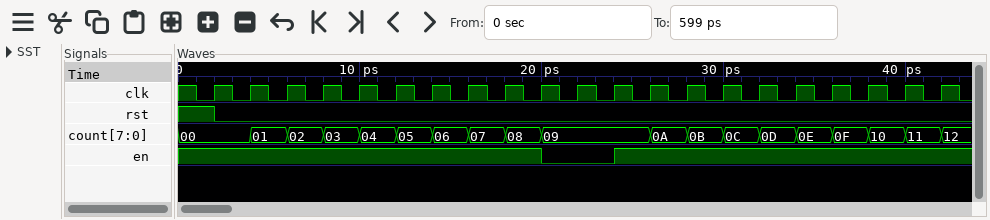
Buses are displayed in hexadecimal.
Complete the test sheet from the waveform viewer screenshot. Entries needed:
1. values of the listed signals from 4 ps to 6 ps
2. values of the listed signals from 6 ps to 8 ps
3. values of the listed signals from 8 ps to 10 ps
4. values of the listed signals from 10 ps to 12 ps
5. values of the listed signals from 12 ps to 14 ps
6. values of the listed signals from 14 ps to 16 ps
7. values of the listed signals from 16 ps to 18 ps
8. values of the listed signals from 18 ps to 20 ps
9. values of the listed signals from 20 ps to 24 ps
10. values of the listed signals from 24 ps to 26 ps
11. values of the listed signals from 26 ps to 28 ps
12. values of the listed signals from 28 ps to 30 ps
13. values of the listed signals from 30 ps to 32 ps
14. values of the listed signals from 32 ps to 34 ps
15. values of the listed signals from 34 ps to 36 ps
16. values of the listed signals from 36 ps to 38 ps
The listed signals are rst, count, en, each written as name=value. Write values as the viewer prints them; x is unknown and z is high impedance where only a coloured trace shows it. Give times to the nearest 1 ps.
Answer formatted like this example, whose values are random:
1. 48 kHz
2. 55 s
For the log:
1. rst=0, count=01, en=1
2. rst=0, count=02, en=1
3. rst=0, count=03, en=1
4. rst=0, count=04, en=1
5. rst=0, count=05, en=1
6. rst=0, count=06, en=1
7. rst=0, count=07, en=1
8. rst=0, count=08, en=1
9. rst=0, count=09, en=0
10. rst=0, count=09, en=1
11. rst=0, count=0A, en=1
12. rst=0, count=0B, en=1
13. rst=0, count=0C, en=1
14. rst=0, count=0D, en=1
15. rst=0, count=0E, en=1
16. rst=0, count=0F, en=1
